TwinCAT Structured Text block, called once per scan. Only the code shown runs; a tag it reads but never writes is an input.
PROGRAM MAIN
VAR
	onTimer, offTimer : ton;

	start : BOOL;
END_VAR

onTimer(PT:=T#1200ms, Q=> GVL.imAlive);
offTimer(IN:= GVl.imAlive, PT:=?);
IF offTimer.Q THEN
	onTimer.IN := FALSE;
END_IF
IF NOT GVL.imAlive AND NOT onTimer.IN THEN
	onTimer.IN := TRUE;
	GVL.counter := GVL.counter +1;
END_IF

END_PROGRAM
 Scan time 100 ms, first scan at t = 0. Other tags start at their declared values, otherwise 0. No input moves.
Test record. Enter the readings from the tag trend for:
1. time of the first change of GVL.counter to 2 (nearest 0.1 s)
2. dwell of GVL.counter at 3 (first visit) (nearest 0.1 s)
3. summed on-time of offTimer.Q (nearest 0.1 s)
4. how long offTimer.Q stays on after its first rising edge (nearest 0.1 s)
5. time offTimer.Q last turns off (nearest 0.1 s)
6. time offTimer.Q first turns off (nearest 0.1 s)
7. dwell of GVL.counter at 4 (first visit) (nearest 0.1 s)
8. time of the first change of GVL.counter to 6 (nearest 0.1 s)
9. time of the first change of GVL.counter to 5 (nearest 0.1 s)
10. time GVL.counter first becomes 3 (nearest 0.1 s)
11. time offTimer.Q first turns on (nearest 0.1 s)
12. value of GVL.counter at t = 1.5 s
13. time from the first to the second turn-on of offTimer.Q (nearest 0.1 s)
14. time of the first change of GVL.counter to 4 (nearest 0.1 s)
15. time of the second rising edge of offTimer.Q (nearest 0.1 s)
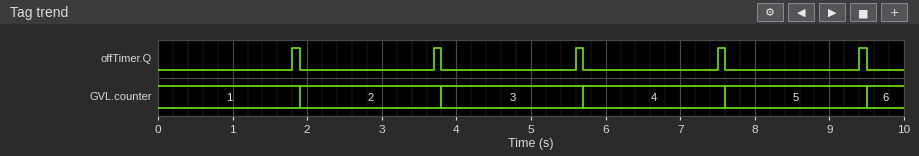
1.9 s
1.9 s
0.5 s
0.1 s
9.5 s
1.9 s
1.9 s
9.5 s
7.6 s
3.8 s
1.8 s
1
1.9 s
5.7 s
3.7 s
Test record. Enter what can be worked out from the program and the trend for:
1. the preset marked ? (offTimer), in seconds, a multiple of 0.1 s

0.5 s
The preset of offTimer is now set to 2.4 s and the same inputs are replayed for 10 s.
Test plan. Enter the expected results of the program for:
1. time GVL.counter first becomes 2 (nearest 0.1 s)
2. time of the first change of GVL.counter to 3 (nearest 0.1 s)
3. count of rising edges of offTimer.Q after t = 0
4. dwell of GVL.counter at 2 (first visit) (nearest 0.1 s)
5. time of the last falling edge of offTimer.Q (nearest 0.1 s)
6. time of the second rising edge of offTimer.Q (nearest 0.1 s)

3.8 s
7.6 s
2
3.8 s
7.6 s
7.5 s
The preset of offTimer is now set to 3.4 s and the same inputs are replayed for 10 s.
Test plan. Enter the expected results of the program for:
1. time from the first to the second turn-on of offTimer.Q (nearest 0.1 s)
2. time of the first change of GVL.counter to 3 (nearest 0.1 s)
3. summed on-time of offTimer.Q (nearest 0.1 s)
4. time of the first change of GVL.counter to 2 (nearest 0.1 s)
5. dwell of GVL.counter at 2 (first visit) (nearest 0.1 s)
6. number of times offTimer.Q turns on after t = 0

4.8 s
9.6 s
0.2 s
4.8 s
4.8 s
2
